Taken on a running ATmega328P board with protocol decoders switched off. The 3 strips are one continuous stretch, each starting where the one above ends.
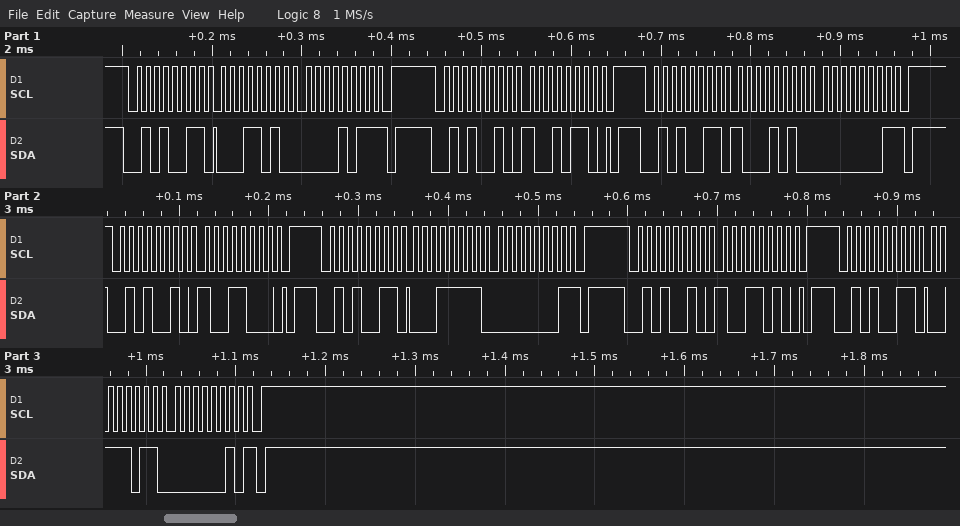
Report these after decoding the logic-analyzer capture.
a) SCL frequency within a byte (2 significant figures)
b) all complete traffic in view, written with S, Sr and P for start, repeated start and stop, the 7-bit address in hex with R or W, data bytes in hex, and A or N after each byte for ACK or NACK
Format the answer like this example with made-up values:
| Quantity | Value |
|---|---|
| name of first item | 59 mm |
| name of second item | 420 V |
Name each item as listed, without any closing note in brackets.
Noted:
| Quantity | Value |
|---|---|
| SCL frequency within a byte | 100 kHz |
| all complete traffic in view, written with S, Sr and P for start, repeated start and stop, the 7-bit address in hex with R or W, data bytes in hex, and A or N after each byte for ACK or NACK | S 29R A 1A A 0B N P S 29W A 96 A P S 29R A 8A A 01 N P S 29W A 98 A P S 29R A 1F A 01 N P S 29W A 9A A P S 29R A 3B A 02 N P |
